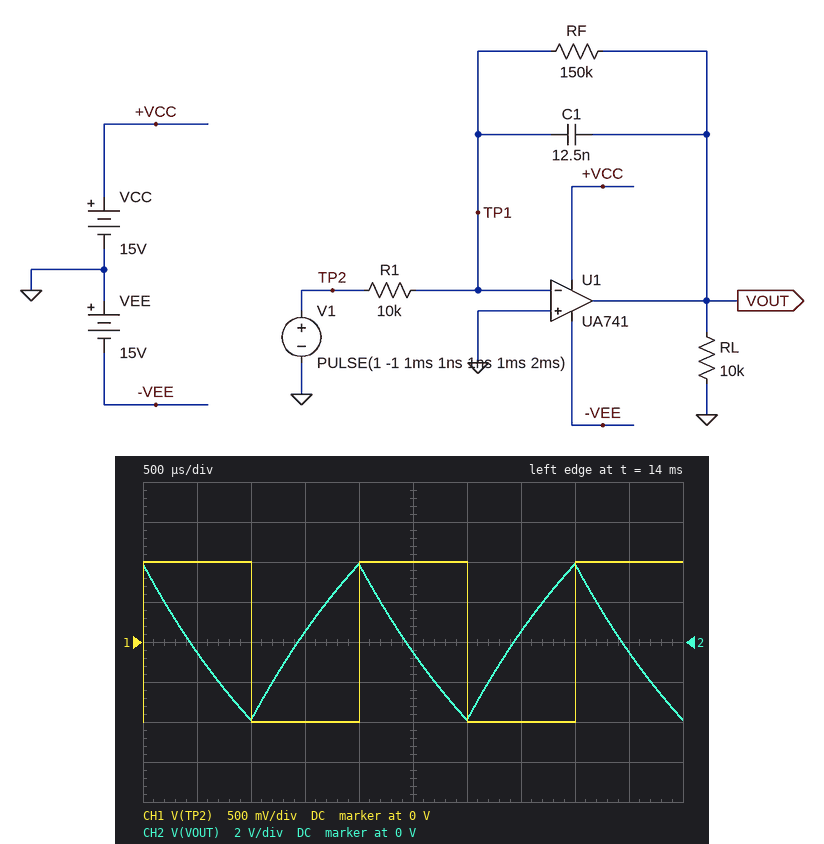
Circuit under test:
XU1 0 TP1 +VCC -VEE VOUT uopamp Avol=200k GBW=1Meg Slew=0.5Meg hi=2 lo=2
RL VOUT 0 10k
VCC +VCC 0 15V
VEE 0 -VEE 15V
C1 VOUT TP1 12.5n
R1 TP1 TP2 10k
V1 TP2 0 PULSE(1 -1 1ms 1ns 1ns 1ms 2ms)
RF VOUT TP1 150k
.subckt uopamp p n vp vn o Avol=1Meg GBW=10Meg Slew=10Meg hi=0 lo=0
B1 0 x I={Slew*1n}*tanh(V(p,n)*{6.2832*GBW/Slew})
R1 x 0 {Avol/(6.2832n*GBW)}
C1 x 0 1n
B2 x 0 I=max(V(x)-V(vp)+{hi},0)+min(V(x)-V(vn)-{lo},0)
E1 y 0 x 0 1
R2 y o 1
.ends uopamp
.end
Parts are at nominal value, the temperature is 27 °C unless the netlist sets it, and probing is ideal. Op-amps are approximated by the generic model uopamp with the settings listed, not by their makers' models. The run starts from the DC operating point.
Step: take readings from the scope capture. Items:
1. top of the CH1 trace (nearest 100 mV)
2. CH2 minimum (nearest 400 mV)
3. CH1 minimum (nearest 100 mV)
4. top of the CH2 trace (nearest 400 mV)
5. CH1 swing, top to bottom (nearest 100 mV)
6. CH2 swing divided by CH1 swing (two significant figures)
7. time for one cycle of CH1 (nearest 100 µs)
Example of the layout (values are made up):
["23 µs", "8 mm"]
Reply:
["1.0 V", "-4.0 V", "-1.0 V", "4.0 V", "2.0 V", "3.9", "2.0 ms"]
